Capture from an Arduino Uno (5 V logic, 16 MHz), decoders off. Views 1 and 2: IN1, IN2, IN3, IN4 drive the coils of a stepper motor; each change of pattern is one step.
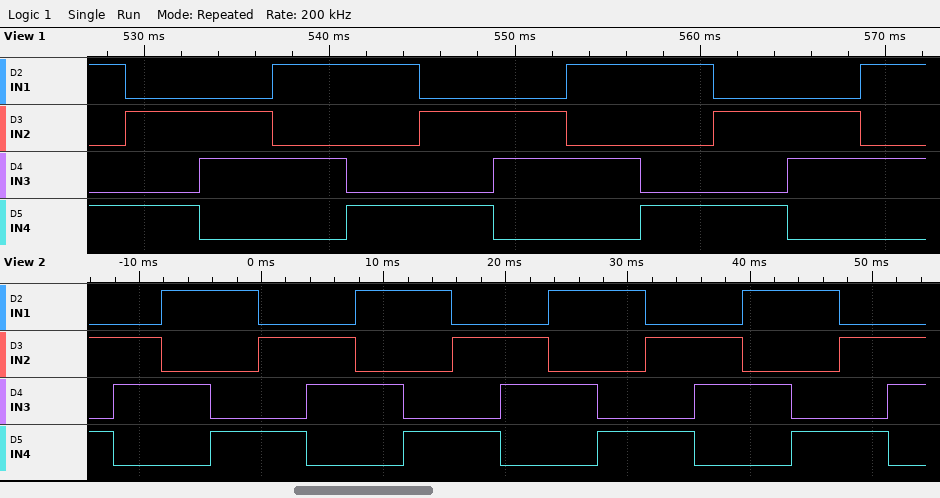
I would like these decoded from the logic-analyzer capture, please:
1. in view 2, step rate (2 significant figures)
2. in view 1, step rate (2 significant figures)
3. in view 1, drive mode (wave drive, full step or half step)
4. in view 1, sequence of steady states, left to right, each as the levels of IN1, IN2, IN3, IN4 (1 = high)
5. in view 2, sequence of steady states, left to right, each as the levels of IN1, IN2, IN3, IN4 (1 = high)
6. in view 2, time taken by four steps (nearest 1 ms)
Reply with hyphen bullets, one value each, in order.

- 250 steps/s
- 250 steps/s
- full step
- 1001 0101 0110 1010 1001 0101 0110 1010 1001 0101 0110 1010
- 0101 0110 1010 1001 0101 0110 1010 1001 0101 0110 1010 1001 0101 0110 1010 1001 0101 0110
- 16 ms
